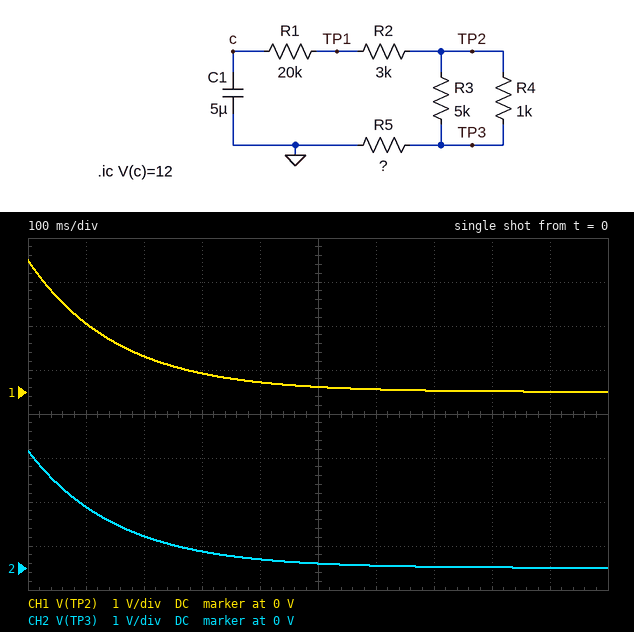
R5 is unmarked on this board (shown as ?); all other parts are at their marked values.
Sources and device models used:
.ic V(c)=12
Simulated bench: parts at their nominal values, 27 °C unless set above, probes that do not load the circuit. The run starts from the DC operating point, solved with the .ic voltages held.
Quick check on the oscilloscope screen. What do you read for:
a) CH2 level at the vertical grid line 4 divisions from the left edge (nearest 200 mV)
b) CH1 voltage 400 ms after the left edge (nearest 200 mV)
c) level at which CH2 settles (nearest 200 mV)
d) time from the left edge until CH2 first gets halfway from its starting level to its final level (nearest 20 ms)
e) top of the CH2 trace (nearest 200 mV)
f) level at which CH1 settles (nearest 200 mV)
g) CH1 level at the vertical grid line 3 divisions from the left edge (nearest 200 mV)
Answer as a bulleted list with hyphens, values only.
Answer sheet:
- 200 mV
- 200 mV
- 0 V
- 100 ms
- 2.6 V
- 0 V
- 400 mV
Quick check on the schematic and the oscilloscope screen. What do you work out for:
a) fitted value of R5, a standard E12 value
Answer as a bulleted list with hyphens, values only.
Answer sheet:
- 6.8 kΩ
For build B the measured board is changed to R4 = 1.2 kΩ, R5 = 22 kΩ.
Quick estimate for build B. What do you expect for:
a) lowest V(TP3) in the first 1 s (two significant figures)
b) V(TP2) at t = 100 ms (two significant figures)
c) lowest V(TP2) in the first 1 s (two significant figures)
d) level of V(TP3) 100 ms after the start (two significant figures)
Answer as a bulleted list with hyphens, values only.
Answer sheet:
- 74 mV
- 3.9 V
- 77 mV
- 3.7 V
